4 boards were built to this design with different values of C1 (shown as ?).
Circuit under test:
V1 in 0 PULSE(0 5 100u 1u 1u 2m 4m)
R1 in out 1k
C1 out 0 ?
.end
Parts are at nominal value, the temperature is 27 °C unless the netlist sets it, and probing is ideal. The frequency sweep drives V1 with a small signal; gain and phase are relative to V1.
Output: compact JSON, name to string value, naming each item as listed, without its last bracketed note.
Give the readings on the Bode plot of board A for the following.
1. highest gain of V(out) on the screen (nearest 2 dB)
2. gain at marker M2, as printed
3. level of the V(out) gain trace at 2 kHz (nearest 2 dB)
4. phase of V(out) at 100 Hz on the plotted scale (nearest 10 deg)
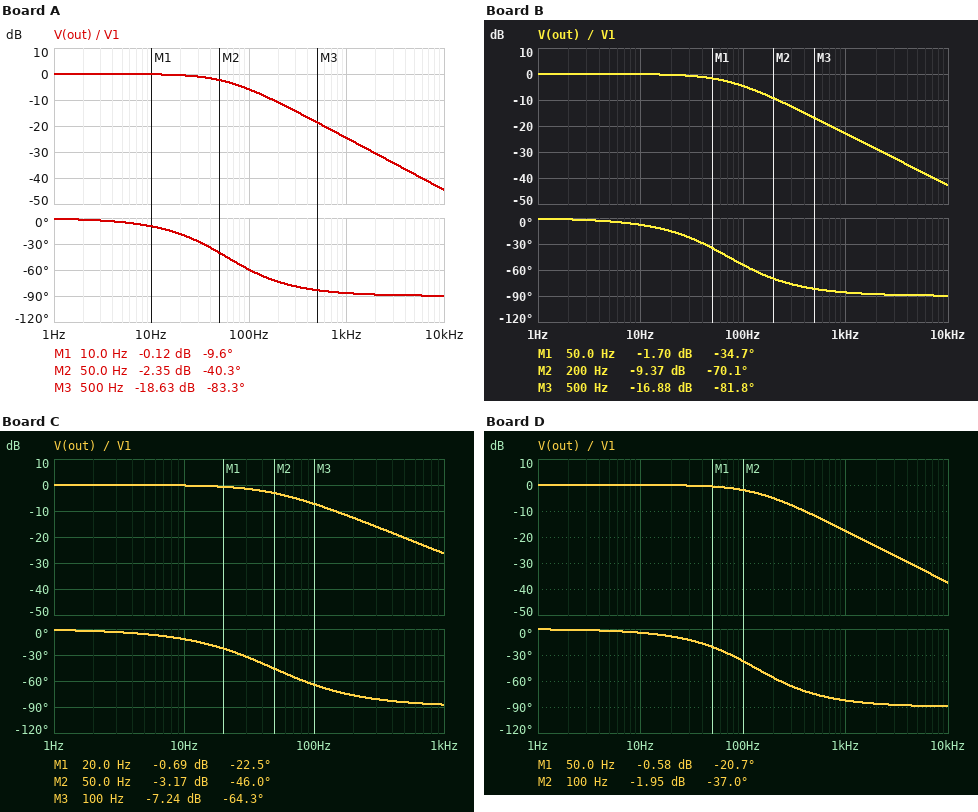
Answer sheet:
{"highest gain of V(out) on the screen": "0 dB", "gain at marker M2, as printed": "-2.35 dB", "level of the V(out) gain trace at 2 kHz": "-30 dB", "phase of V(out) at 100 Hz on the plotted scale": "-60 deg"}
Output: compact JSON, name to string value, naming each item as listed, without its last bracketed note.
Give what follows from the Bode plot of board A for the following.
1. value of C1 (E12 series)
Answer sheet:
{"value of C1": "2.7 µF"}
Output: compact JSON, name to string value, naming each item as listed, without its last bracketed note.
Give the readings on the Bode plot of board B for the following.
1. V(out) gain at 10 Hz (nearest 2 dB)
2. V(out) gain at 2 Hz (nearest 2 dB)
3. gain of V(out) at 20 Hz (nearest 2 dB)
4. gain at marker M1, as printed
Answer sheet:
{"V(out) gain at 10 Hz": "0 dB", "V(out) gain at 2 Hz": "0 dB", "gain of V(out) at 20 Hz": "0 dB", "gain at marker M1, as printed": "-1.70 dB"}
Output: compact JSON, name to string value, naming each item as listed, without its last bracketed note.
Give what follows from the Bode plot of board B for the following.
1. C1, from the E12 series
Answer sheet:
{"C1, from the E12 series": "2.2 µF"}
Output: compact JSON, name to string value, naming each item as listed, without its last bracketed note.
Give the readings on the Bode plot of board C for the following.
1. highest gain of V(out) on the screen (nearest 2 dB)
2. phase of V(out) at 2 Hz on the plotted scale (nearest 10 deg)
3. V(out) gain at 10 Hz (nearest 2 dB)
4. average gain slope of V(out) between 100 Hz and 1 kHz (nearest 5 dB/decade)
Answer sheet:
{"highest gain of V(out) on the screen": "0 dB", "phase of V(out) at 2 Hz on the plotted scale": "0 deg", "V(out) gain at 10 Hz": "0 dB", "average gain slope of V(out) between 100 Hz and 1 kHz": "-20 dB/decade"}
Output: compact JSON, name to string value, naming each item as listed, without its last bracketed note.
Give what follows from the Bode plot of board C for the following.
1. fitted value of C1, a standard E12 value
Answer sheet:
{"fitted value of C1, a standard E12 value": "3.3 µF"}
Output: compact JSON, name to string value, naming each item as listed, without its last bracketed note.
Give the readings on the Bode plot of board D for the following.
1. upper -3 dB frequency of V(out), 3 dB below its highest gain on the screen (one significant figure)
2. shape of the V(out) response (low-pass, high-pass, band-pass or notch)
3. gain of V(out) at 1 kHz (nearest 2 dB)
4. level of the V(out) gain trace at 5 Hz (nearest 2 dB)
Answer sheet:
{"upper -3 dB frequency of V(out), 3 dB below its highest gain on the screen": "100 Hz", "shape of the V(out) response": "low-pass", "gain of V(out) at 1 kHz": "-18 dB", "level of the V(out) gain trace at 5 Hz": "0 dB"}
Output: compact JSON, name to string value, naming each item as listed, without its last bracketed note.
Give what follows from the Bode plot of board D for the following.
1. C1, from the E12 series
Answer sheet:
{"C1, from the E12 series": "1.2 µF"}
